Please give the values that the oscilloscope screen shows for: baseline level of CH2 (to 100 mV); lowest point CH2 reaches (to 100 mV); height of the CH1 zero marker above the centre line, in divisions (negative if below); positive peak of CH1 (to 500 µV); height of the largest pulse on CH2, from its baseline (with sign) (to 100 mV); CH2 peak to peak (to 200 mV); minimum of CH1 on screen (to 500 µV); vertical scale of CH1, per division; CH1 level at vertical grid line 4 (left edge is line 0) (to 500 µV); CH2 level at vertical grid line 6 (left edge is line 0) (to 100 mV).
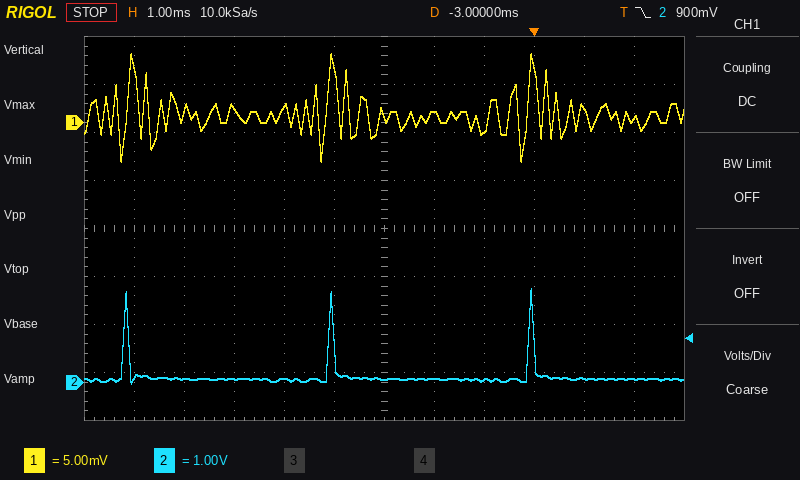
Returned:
100 mV
0.0 V
+2.2 div
7.0 mV
+1.9 V
2.0 V
-4.0 mV
5 mV
1.5 mV
100 mV
